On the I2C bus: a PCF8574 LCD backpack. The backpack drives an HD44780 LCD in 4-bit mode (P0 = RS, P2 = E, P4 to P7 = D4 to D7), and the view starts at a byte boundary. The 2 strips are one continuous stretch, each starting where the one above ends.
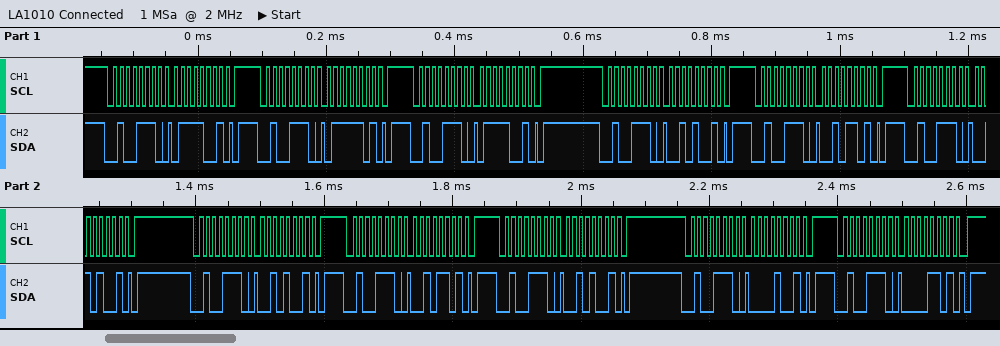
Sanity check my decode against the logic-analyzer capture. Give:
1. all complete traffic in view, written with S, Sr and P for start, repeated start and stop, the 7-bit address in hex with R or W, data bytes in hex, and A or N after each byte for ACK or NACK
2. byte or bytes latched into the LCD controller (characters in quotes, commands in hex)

S 27W A 79 A P S 27W A 7D A P S 27W A 79 A P S 27W A 29 A P S 27W A 2D A P S 27W A 29 A P S 27W A 29 A P S 27W A 2D A P S 27W A 29 A P S 27W A 09 A P S 27W A 0D A P
'r'
